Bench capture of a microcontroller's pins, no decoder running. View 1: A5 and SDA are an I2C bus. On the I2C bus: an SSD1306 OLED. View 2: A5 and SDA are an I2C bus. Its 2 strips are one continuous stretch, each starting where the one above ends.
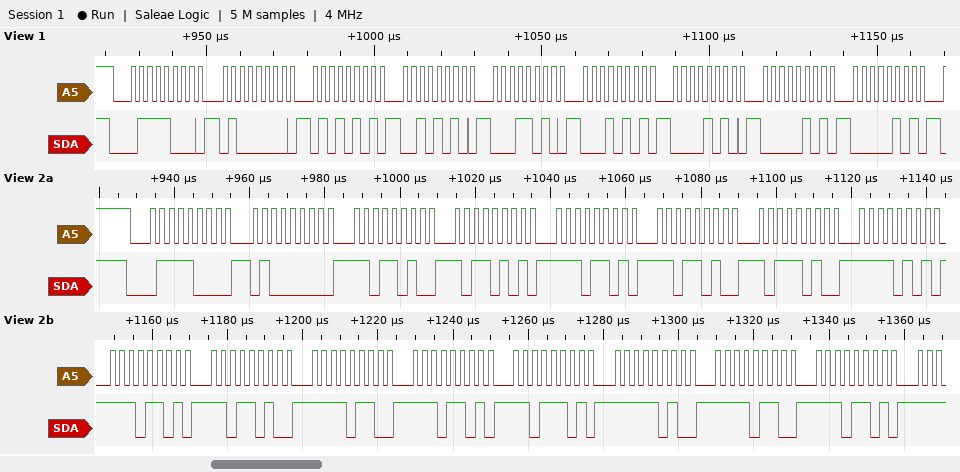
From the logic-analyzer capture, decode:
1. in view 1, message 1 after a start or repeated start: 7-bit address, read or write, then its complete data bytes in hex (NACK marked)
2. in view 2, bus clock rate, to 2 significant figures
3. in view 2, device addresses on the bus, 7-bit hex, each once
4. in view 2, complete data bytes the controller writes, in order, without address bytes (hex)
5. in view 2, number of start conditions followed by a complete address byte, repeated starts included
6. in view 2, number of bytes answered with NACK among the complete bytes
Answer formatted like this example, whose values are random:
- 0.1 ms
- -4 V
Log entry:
- 0x3C write: 40 55 2A 1A 15 0A 05 05
- 400 kHz
- 0x3C
- 40 DA B5 ED DA BA F5 ED DA F6 ED DD FA F6 ED
- 1
- 0
